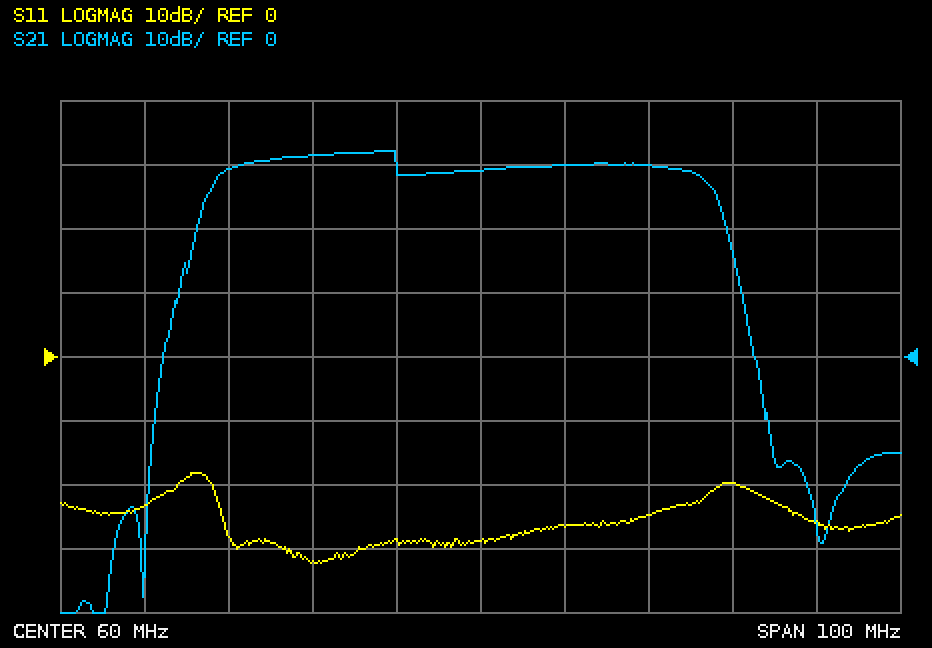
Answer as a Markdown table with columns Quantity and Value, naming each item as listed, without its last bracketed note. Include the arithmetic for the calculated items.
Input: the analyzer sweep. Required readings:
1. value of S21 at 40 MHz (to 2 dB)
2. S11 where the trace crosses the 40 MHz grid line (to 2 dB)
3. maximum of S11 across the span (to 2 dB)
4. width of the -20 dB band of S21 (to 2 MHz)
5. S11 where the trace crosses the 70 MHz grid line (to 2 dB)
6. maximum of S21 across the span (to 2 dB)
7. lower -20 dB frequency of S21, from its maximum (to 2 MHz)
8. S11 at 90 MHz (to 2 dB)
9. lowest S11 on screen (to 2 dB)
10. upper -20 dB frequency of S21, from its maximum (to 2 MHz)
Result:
| Quantity | Value |
|---|---|
| value of S21 at 40 MHz | 32 dB |
| S11 where the trace crosses the 40 MHz grid line | -32 dB |
| maximum of S11 across the span | -18 dB |
| width of the -20 dB band of S21 | 90 MHz − 24 MHz = 66 MHz |
| S11 where the trace crosses the 70 MHz grid line | -26 dB |
| maximum of S21 across the span | 32 dB |
| lower -20 dB frequency of S21, from its maximum | 24 MHz |
| S11 at 90 MHz | -20 dB |
| lowest S11 on screen | -32 dB |
| upper -20 dB frequency of S21, from its maximum | 90 MHz |
